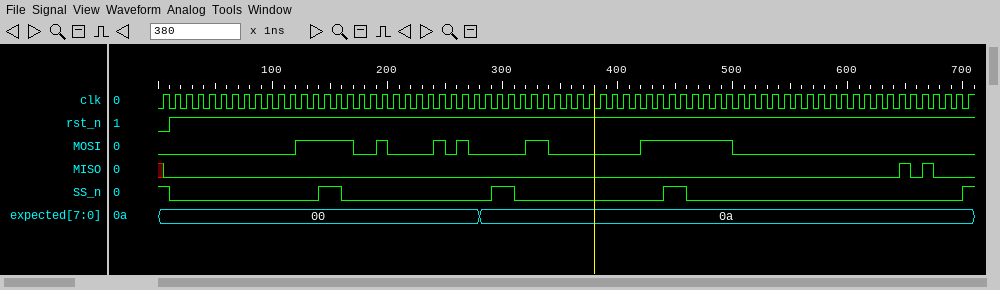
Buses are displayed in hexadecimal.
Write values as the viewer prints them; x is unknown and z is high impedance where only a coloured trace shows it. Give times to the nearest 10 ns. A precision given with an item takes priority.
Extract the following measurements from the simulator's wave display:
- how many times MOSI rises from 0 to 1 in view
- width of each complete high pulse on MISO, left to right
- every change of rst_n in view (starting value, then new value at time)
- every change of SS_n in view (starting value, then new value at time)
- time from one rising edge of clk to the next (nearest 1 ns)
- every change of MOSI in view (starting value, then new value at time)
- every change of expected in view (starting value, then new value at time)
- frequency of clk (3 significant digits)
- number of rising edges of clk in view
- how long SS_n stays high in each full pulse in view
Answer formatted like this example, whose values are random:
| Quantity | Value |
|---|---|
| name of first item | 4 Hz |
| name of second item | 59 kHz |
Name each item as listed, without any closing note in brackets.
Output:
| Quantity | Value |
|---|---|
| how many times MOSI rises from 0 to 1 in view | 6 |
| width of each complete high pulse on MISO, left to right | 10 ns, 10 ns |
| every change of rst_n in view | 0, 1 at 10 ns |
| every change of SS_n in view | 1, 0 at 10 ns, 1 at 140 ns, 0 at 160 ns, 1 at 290 ns, 0 at 310 ns, 1 at 440 ns, 0 at 460 ns, 1 at 700 ns |
| time from one rising edge of clk to the next | 10 ns |
| every change of MOSI in view | 0, 1 at 120 ns, 0 at 170 ns, 1 at 190 ns, 0 at 200 ns, 1 at 240 ns, 0 at 250 ns, 1 at 260 ns, 0 at 270 ns, 1 at 320 ns, 0 at 340 ns, 1 at 420 ns, 0 at 500 ns |
| every change of expected in view | 00, 0a at 280 ns |
| frequency of clk | 100 MHz |
| number of rising edges of clk in view | 71 |
| how long SS_n stays high in each full pulse in view | 20 ns, 20 ns, 20 ns |
